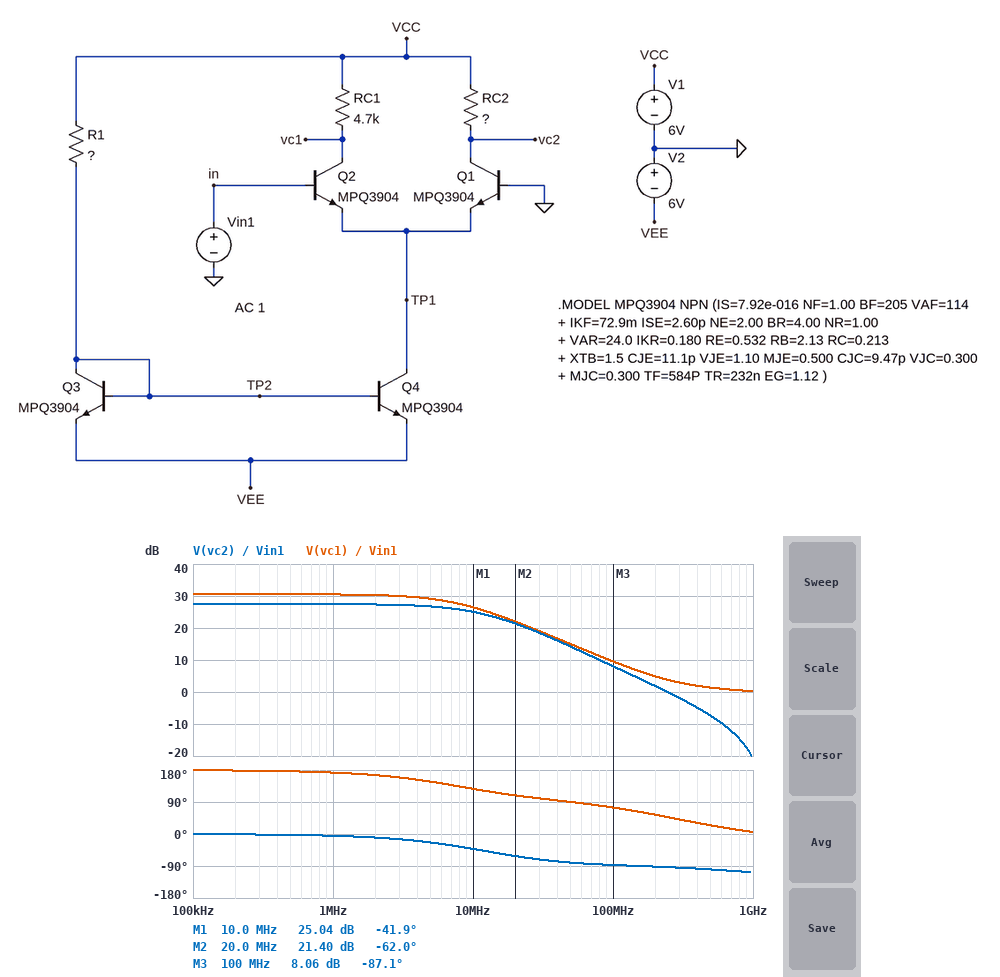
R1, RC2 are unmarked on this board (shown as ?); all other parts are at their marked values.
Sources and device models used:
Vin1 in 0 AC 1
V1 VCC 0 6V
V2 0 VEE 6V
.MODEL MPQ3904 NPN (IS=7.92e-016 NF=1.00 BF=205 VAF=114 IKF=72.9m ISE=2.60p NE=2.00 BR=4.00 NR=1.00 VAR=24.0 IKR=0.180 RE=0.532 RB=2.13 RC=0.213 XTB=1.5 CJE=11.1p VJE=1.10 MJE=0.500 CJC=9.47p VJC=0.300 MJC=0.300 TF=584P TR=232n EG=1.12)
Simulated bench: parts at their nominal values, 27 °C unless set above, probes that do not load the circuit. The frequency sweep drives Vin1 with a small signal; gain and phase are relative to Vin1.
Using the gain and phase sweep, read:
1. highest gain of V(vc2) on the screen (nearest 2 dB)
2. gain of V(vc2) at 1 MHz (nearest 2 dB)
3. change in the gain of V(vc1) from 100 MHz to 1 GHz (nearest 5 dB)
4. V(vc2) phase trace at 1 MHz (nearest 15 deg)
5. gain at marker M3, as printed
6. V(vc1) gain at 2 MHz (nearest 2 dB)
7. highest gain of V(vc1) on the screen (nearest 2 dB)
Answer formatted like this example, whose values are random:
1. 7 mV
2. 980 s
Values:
1. 28 dB
2. 28 dB
3. -10 dB
4. 0 deg
5. 8.06 dB
6. 30 dB
7. 30 dB
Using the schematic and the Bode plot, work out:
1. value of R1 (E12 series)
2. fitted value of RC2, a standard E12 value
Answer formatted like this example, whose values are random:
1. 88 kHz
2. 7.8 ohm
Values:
1. 15 kΩ
2. 3.3 kΩ
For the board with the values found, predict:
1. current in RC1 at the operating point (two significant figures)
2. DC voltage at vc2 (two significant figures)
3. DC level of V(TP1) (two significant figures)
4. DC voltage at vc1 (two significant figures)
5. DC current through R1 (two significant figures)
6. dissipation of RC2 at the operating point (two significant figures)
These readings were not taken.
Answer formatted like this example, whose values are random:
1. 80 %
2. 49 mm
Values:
1. 380 µA
2. 4.7 V
3. -700 mV
4. 4.2 V
5. 750 µA
6. 480 µW
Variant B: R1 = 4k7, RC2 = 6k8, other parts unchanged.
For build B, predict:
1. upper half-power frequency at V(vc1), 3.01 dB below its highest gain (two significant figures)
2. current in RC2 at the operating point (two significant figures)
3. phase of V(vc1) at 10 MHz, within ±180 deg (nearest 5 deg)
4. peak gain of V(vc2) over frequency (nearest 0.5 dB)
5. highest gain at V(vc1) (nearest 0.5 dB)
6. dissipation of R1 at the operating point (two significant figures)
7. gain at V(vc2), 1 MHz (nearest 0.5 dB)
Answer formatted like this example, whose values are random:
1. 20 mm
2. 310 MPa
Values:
1. 2.5 MHz
2. 980 µA
3. 100 deg
4. 9.0 dB
5. 39.0 dB
6. 27 mW
7. 1.5 dB
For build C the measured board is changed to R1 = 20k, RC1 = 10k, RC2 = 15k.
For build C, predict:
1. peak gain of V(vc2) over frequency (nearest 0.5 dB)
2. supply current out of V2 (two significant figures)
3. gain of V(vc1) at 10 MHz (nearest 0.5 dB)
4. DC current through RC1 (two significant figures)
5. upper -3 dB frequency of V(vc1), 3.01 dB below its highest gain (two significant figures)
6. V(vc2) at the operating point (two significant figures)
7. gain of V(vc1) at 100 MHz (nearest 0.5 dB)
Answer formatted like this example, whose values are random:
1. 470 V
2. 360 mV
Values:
1. 38.0 dB
2. 1.1 mA
3. 25.0 dB
4. 290 µA
5. 3.5 MHz
6. 1.7 V
7. 7.0 dB
